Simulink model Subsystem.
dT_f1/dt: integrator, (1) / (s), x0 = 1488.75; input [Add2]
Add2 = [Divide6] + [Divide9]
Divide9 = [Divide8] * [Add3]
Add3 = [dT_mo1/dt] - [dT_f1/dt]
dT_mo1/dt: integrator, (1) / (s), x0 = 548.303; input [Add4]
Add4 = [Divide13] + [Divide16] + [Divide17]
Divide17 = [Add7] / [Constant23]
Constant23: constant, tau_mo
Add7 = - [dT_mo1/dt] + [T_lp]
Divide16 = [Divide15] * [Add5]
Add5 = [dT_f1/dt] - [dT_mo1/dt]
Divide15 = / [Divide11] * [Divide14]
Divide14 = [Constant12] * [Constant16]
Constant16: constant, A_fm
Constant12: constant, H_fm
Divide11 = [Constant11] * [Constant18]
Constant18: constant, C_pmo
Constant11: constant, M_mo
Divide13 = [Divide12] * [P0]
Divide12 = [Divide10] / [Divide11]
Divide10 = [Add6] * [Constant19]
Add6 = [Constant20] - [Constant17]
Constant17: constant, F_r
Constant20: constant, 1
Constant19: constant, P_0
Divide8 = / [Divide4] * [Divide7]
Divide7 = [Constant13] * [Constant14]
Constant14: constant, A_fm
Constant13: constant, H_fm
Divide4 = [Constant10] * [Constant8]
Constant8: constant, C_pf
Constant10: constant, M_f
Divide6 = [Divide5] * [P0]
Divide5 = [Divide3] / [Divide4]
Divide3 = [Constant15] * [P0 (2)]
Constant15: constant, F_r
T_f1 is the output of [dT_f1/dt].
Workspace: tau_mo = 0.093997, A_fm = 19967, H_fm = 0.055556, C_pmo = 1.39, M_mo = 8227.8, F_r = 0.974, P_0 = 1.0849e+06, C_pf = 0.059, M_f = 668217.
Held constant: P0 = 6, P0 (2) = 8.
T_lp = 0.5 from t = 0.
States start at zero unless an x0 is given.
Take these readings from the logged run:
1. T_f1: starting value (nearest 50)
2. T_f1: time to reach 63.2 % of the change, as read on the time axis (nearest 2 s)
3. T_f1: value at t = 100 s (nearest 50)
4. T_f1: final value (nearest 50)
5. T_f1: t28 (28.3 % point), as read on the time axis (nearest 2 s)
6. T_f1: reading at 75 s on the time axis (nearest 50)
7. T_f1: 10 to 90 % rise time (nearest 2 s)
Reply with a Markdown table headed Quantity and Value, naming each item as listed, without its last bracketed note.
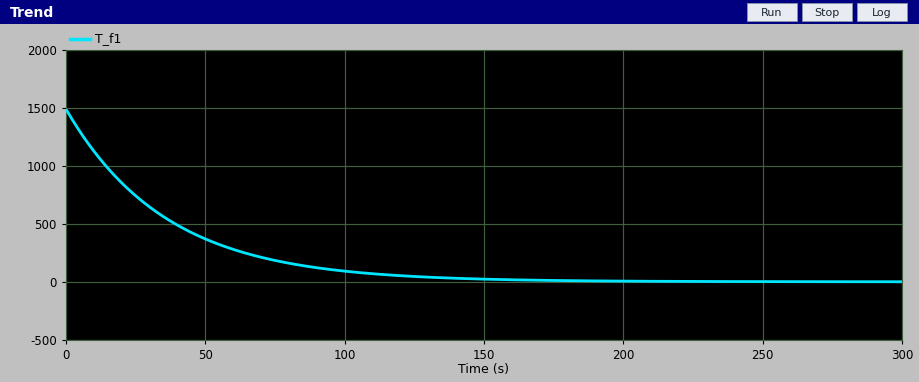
| Quantity | Value |
|---|---|
| T_f1: starting value | 1500 |
| T_f1: time to reach 63.2 % of the change, as read on the time axis | 36 s |
| T_f1: value at t = 100 s | 100 |
| T_f1: final value | 0 |
| T_f1: t28 (28.3 % point), as read on the time axis | 12 s |
| T_f1: reading at 75 s on the time axis | 200 |
| T_f1: 10 to 90 % rise time | 78 s |
